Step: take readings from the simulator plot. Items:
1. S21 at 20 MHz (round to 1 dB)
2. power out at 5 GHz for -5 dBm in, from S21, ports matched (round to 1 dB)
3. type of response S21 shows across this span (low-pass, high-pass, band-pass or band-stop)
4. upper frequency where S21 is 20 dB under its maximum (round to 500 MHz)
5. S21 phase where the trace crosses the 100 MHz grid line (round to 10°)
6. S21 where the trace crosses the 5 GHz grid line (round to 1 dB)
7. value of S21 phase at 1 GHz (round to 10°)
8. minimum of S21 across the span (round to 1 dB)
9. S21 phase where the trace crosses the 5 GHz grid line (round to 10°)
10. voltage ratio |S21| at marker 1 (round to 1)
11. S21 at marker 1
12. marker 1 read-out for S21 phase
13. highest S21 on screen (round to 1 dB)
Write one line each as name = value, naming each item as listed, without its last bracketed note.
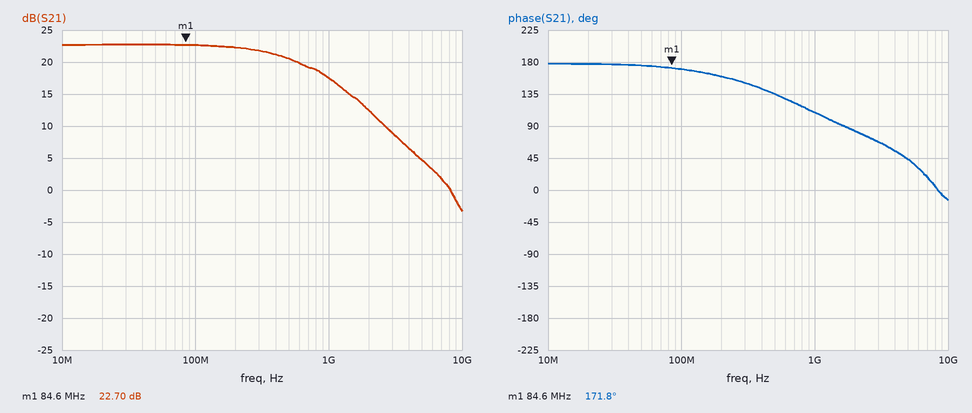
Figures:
S21 at 20 MHz = 23 dB
power out at 5 GHz for -5 dBm in, from S21, ports matched = 0 dBm
type of response S21 shows across this span = low-pass
upper frequency where S21 is 20 dB under its maximum = 6.5 GHz
S21 phase where the trace crosses the 100 MHz grid line = 170°
S21 where the trace crosses the 5 GHz grid line = 5 dB
value of S21 phase at 1 GHz = 110°
minimum of S21 across the span = -3 dB
S21 phase where the trace crosses the 5 GHz grid line = 40°
voltage ratio |S21| at marker 1 = 14
S21 at marker 1 = 22.70 dB
marker 1 read-out for S21 phase = 171.8°
highest S21 on screen = 23 dB
